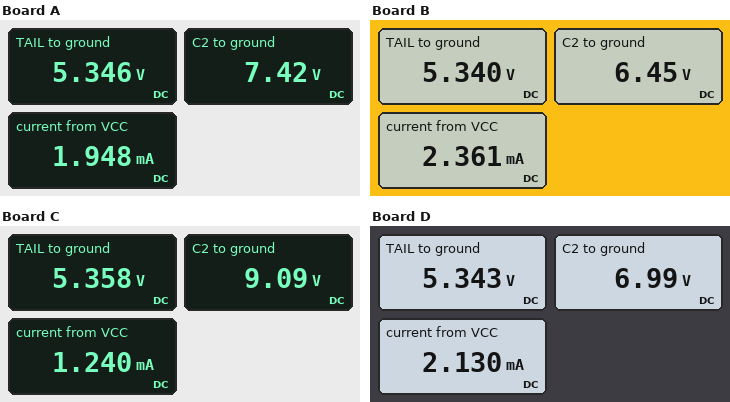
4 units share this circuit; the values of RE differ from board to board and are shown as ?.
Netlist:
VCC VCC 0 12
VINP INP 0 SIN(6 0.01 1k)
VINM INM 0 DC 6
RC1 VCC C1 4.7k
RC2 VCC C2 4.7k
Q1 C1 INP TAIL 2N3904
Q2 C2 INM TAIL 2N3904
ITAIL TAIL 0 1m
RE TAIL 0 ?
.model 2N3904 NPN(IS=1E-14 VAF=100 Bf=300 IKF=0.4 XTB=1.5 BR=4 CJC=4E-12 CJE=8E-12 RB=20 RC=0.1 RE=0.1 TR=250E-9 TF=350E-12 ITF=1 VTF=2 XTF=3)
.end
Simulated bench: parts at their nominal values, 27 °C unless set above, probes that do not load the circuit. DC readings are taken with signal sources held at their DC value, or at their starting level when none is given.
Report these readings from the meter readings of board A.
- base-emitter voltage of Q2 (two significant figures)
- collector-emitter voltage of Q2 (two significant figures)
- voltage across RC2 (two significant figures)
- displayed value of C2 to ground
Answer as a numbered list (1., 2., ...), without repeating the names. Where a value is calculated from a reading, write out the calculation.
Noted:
1. 6 V - 5.346 V = 650 mV
2. 7.42 V - 5.346 V = 2.1 V
3. 12 V - 7.42 V = 4.6 V
4. 7.42 V
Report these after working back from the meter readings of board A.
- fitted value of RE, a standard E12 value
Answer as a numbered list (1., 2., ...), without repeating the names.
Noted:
1. 5.6 kΩ
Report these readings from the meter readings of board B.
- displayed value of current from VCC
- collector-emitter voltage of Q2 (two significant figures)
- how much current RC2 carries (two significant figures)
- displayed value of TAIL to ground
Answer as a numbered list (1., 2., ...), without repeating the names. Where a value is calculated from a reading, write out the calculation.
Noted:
1. 2.361 mA
2. 6.45 V - 5.34 V = 1.1 V
3. (12 V - 6.45 V) / 4.7 kΩ = 1.2 mA
4. 5.340 V
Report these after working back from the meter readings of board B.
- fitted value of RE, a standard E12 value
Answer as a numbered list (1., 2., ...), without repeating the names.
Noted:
1. 3.9 kΩ
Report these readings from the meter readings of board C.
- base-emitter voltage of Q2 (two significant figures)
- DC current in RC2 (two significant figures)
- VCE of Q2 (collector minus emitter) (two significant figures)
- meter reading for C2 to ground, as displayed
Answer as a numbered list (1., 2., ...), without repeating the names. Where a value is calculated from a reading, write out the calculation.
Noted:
1. 6 V - 5.358 V = 640 mV
2. (12 V - 9.09 V) / 4.7 kΩ = 620 µA
3. 9.09 V - 5.358 V = 3.7 V
4. 9.09 V
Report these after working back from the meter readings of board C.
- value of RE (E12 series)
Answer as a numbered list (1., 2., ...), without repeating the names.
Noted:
1. 22 kΩ
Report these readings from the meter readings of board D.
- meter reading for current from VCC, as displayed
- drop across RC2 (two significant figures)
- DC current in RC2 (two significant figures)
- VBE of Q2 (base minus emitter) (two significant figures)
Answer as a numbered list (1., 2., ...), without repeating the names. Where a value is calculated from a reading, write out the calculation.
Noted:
1. 2.130 mA
2. 12 V - 6.99 V = 5.0 V
3. (12 V - 6.99 V) / 4.7 kΩ = 1.1 mA
4. 6 V - 5.343 V = 660 mV
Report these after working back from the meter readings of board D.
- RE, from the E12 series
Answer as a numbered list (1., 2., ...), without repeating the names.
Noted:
1. 4.7 kΩ
